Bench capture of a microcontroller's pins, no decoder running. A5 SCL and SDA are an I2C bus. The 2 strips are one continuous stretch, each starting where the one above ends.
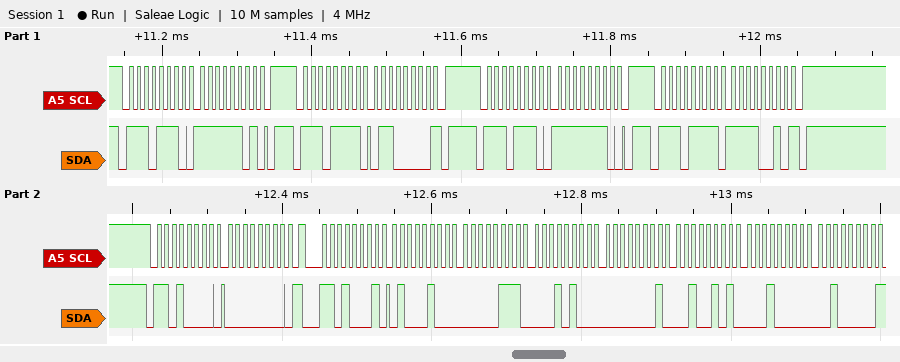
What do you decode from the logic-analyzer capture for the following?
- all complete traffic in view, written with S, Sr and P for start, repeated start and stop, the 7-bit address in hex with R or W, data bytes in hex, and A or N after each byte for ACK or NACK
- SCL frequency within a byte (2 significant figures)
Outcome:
S 77W A FD A P S 77R A 60 N P S 77W A FE A P S 77R A F2 N P S 68W A 00 A Sr 68R A 44 A 07 A 14 A 01 A 25 A 10 A 20 N
100 kHz
